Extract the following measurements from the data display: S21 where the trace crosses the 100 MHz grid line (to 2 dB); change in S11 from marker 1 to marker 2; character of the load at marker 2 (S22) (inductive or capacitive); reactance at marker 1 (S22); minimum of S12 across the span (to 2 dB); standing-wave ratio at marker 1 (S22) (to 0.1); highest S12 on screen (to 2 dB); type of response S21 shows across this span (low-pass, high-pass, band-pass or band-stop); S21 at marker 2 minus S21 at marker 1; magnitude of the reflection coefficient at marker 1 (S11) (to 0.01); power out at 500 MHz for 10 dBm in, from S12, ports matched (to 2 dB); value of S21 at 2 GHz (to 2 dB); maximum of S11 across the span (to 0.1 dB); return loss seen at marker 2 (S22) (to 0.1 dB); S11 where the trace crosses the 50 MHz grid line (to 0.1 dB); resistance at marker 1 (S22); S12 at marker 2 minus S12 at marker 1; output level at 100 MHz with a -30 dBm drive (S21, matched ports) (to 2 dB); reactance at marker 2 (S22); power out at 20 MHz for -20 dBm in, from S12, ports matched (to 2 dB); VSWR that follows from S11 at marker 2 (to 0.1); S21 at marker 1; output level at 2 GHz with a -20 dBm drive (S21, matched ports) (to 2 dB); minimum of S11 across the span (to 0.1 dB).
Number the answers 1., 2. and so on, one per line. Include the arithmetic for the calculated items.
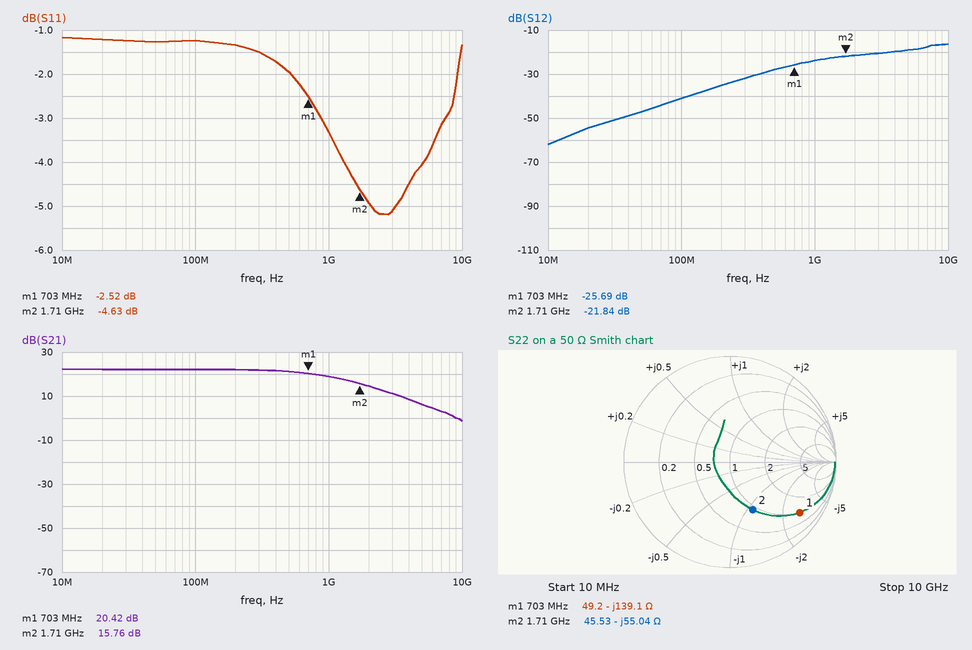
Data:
1. 22 dB
2. -4.63 − (-2.52) = -2.11 dB
3. capacitive
4. -139.1 Ω
5. -62 dB
6. 9.8
7. -16 dB
8. low-pass
9. 15.76 − (20.42) = -4.66 dB
10. 10^(-2.52/20) ≈ 0.75
11. 10 dBm + (-28 dB) = -18 dBm
12. 14 dB
13. -1.2 dB
14. 6.0 dB
15. -1.3 dB
16. 49.2 Ω
17. -21.84 − (-25.69) = 3.85 dB
18. -30 dBm + (22 dB) = -8 dBm
19. -55.04 Ω
20. -20 dBm + (-54 dB) = -74 dBm
21. (1 + 0.5868)/(1 − 0.5868) ≈ 3.8
22. 20.42 dB
23. -20 dBm + (14 dB) = -6 dBm
24. -5.2 dB
